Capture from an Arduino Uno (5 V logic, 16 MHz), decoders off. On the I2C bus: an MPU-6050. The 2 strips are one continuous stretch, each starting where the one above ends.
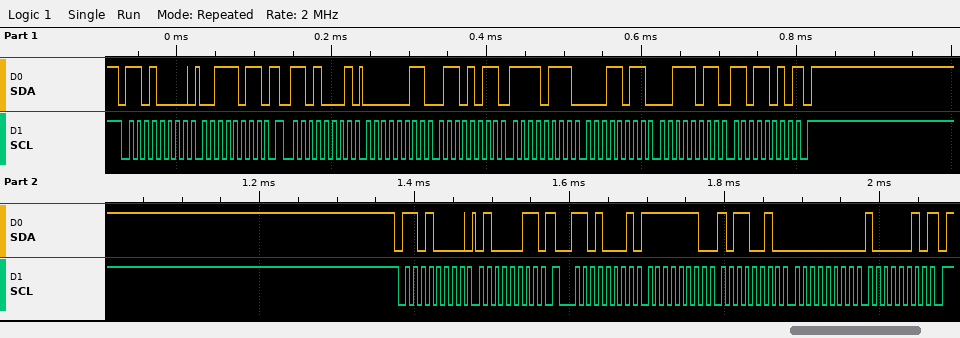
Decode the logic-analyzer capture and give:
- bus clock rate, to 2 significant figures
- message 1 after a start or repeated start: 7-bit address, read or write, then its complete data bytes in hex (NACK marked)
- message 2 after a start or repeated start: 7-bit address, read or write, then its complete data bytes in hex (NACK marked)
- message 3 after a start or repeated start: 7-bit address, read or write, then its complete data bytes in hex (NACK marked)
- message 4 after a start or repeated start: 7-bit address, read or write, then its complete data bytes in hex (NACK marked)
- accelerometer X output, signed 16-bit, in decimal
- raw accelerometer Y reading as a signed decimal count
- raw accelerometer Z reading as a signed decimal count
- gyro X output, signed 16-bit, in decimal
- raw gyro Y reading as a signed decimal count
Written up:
100 kHz
0x68 write: 3B
0x68 read: 03 6B F7 1B 3B DA NACK
0x68 write: 43
0x68 read: FE B2 00 82 NACK
875
-2277
15322
-334
130
